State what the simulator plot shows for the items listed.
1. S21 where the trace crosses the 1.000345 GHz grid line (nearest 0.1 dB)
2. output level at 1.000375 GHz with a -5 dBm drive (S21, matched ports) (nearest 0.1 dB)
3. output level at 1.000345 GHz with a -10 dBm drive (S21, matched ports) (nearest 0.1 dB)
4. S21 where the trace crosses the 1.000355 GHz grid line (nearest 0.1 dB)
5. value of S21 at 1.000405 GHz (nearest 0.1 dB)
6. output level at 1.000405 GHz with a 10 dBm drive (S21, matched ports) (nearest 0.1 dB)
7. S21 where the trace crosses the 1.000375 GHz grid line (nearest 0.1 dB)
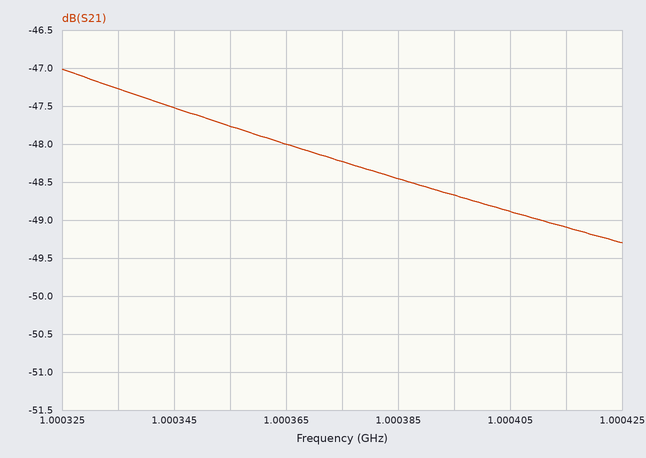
-47.5 dB
-53.2 dBm
-57.5 dBm
-47.8 dB
-48.9 dB
-38.9 dBm
-48.2 dB
